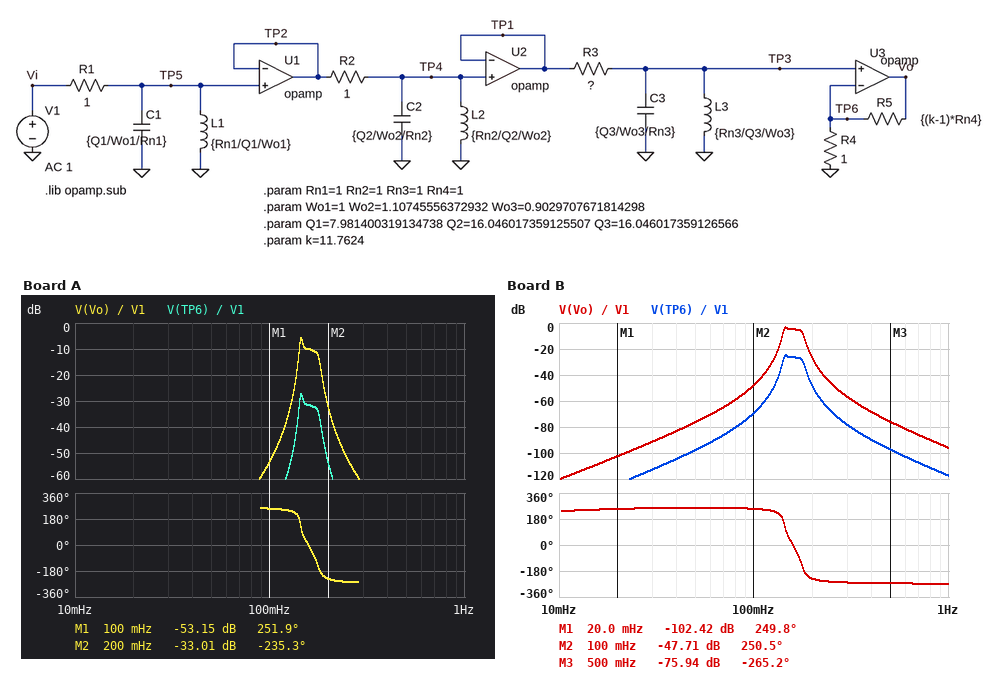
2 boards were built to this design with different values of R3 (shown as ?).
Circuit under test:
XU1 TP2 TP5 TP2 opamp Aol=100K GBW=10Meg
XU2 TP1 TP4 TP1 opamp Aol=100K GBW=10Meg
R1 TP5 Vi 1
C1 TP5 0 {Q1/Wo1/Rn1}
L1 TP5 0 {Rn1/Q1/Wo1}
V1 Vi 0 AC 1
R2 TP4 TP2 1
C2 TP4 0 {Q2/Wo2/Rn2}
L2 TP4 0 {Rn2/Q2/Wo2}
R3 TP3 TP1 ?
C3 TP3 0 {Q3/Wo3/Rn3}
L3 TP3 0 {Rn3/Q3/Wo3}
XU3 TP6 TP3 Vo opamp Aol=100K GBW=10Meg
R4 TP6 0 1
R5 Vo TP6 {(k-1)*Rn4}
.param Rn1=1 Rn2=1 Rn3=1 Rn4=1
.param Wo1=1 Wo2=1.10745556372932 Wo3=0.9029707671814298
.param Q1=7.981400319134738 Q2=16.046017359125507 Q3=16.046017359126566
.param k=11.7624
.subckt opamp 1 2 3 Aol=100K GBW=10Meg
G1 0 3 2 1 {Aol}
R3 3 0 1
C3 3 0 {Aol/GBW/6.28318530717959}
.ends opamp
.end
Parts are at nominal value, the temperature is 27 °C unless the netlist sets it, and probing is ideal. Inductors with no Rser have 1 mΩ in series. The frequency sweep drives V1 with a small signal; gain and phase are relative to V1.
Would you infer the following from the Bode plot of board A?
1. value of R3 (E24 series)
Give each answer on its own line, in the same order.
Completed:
3 Ω
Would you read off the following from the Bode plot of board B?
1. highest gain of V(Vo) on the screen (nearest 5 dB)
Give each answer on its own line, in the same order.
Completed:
-5 dB
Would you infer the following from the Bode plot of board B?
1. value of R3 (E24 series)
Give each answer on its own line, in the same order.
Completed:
1.6 Ω
